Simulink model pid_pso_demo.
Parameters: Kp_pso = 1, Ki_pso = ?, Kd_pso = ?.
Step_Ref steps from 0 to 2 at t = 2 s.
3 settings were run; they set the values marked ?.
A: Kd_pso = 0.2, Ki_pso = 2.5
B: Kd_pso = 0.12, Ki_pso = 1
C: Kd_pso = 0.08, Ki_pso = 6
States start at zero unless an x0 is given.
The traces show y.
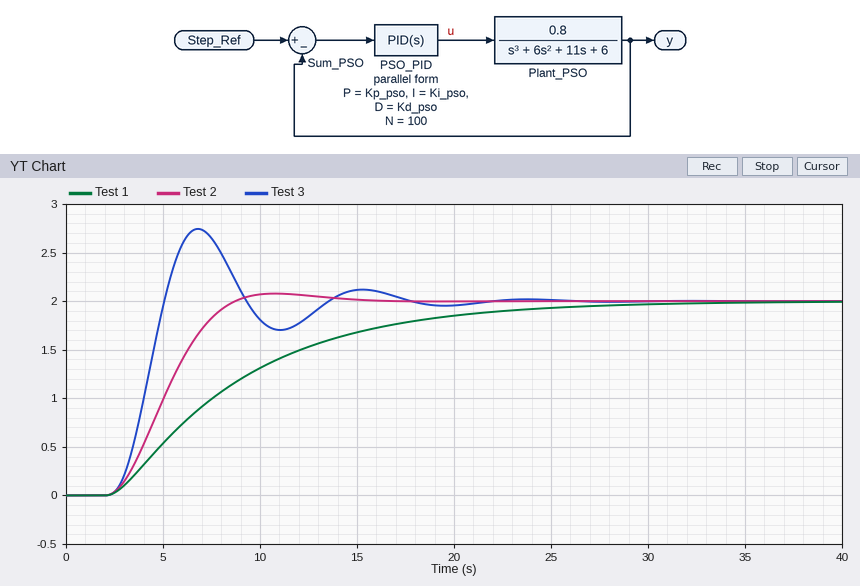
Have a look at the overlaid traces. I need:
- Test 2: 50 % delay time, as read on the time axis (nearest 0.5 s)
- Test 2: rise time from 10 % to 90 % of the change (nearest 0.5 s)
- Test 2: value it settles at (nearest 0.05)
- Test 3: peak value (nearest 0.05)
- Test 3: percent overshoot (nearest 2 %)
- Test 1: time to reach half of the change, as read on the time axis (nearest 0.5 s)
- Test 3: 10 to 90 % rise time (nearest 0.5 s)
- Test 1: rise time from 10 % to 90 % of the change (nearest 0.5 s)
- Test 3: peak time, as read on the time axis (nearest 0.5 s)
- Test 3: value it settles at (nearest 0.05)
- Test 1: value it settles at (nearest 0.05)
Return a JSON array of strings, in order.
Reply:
["5.0 s", "4.0 s", "2.00", "2.75", "38 %", "7.5 s", "2.0 s", "14.5 s", "7.0 s", "2.00", "2.00"]
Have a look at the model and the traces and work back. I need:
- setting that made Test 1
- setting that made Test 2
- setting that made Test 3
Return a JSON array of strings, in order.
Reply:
["B", "A", "C"]
